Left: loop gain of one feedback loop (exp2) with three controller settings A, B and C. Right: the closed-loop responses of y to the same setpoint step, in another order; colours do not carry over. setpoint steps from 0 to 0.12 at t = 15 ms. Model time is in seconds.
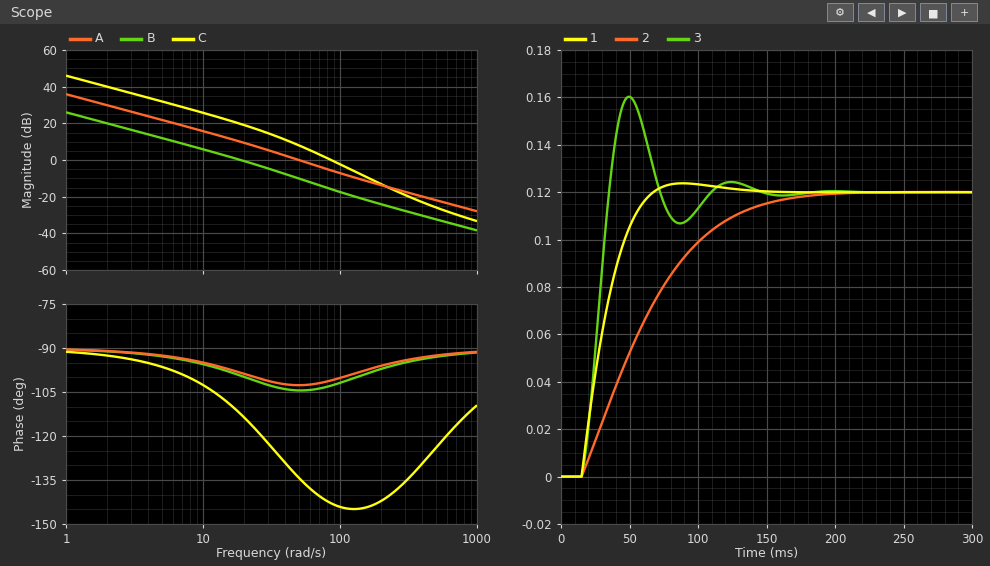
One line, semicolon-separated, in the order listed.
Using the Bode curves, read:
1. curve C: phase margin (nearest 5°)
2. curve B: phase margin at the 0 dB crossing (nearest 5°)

35°; 80°
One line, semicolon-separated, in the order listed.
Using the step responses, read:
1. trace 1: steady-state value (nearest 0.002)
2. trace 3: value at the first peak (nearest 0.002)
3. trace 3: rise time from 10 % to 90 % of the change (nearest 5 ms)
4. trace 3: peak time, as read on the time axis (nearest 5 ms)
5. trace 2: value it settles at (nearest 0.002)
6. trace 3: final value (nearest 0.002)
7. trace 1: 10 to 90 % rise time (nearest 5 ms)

0.120; 0.160; 15 ms; 50 ms; 0.120; 0.120; 35 ms
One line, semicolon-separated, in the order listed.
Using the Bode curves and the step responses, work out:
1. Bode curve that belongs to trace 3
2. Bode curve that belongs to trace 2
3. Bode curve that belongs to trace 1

C; B; A
